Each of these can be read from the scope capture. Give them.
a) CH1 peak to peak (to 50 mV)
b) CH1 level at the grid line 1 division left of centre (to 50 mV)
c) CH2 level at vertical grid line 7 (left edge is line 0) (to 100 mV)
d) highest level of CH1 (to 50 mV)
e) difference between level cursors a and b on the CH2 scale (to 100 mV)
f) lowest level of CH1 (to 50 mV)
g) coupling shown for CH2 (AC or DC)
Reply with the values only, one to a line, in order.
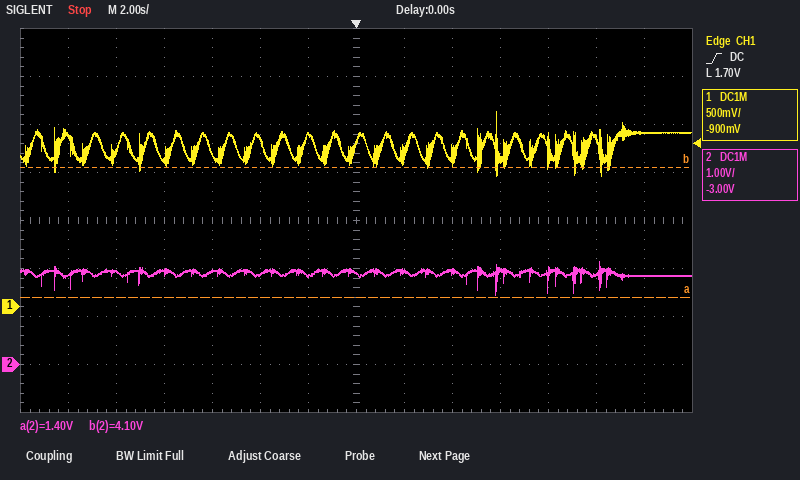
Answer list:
700 mV
1.80 V
1.9 V
2.05 V
2.7 V
1.35 V
DC
